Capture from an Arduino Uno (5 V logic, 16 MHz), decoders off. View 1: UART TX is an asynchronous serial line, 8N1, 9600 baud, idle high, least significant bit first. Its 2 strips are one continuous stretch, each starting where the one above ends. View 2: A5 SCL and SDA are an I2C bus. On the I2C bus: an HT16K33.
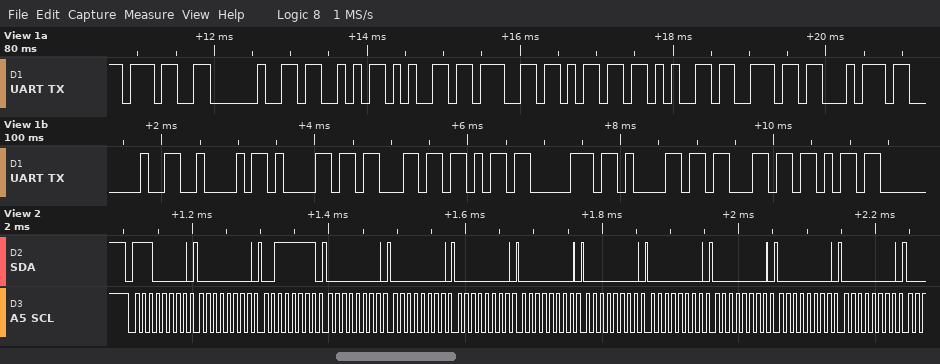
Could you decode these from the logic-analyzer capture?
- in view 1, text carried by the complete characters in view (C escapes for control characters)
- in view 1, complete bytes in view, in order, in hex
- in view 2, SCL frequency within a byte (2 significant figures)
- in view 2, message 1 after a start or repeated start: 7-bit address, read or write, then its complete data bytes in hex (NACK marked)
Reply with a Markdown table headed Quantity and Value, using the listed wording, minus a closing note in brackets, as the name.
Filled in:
| Quantity | Value |
|---|---|
| in view 1, text carried by the complete characters in view | "7 Segment Backpack" |
| in view 1, complete bytes in view, in order, in hex | 37 20 53 65 67 6D 65 6E 74 20 42 61 63 6B 70 61 63 6B |
| in view 2, SCL frequency within a byte | 100 kHz |
| in view 2, message 1 after a start or repeated start: 7-bit address, read or write, then its complete data bytes in hex | 0x70 write: 00 3F 00 00 00 00 00 00 00 00 00 |
